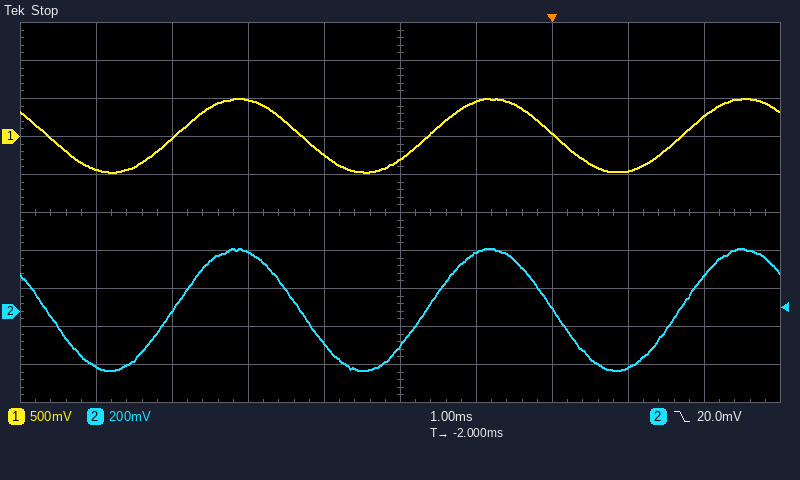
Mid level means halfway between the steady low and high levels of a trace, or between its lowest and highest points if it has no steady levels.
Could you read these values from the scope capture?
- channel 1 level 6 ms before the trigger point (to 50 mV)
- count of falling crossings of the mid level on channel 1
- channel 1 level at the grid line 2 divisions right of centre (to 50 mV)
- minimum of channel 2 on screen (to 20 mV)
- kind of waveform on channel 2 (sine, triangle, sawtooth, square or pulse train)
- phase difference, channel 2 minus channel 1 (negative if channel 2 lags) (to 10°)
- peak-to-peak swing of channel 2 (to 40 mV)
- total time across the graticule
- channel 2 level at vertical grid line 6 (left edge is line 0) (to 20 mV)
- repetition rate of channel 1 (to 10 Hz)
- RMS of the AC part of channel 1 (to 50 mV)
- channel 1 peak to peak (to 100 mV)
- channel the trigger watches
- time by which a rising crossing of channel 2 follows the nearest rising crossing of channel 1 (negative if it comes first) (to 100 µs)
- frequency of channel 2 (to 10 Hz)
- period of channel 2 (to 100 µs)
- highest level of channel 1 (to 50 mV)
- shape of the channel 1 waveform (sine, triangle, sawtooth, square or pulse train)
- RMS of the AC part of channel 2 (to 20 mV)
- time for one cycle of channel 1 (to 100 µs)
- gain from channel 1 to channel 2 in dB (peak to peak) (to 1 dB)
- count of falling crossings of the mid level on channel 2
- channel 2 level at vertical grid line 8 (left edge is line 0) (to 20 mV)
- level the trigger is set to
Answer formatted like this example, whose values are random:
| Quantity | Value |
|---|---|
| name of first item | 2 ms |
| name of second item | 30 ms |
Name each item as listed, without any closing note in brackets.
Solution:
| Quantity | Value |
|---|---|
| channel 1 level 6 ms before the trigger point | -450 mV |
| count of falling crossings of the mid level on channel 1 | 3 |
| channel 1 level at the grid line 2 divisions right of centre | 50 mV |
| minimum of channel 2 on screen | -320 mV |
| kind of waveform on channel 2 | sine |
| phase difference, channel 2 minus channel 1 (negative if channel 2 lags) | 0° |
| peak-to-peak swing of channel 2 | 640 mV |
| total time across the graticule | 10 ms |
| channel 2 level at vertical grid line 6 (left edge is line 0) | 300 mV |
| repetition rate of channel 1 | 300 Hz |
| RMS of the AC part of channel 1 | 350 mV |
| channel 1 peak to peak | 1.00 V |
| channel the trigger watches | channel 2 |
| time by which a rising crossing of channel 2 follows the nearest rising crossing of channel 1 (negative if it comes first) | 0.0 ms |
| frequency of channel 2 | 300 Hz |
| period of channel 2 | 3.3 ms |
| highest level of channel 1 | 500 mV |
| shape of the channel 1 waveform | sine |
| RMS of the AC part of channel 2 | 220 mV |
| time for one cycle of channel 1 | 3.3 ms |
| gain from channel 1 to channel 2 in dB (peak to peak) | -4 dB |
| count of falling crossings of the mid level on channel 2 | 3 |
| channel 2 level at vertical grid line 8 (left edge is line 0) | -300 mV |
| level the trigger is set to | 20.0 mV |
